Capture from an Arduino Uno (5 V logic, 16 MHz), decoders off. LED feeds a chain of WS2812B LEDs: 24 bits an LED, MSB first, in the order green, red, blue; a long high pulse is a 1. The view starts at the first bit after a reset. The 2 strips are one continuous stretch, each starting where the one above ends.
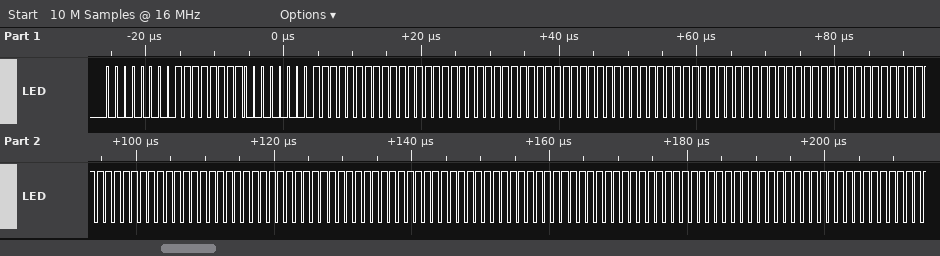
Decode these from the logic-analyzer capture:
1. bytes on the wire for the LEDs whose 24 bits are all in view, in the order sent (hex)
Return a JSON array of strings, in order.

["00 FF 00 FF FF FF FF FF FF FF FF FF FF FF FF FF FF FF FF FF FF FF FF FF"]
